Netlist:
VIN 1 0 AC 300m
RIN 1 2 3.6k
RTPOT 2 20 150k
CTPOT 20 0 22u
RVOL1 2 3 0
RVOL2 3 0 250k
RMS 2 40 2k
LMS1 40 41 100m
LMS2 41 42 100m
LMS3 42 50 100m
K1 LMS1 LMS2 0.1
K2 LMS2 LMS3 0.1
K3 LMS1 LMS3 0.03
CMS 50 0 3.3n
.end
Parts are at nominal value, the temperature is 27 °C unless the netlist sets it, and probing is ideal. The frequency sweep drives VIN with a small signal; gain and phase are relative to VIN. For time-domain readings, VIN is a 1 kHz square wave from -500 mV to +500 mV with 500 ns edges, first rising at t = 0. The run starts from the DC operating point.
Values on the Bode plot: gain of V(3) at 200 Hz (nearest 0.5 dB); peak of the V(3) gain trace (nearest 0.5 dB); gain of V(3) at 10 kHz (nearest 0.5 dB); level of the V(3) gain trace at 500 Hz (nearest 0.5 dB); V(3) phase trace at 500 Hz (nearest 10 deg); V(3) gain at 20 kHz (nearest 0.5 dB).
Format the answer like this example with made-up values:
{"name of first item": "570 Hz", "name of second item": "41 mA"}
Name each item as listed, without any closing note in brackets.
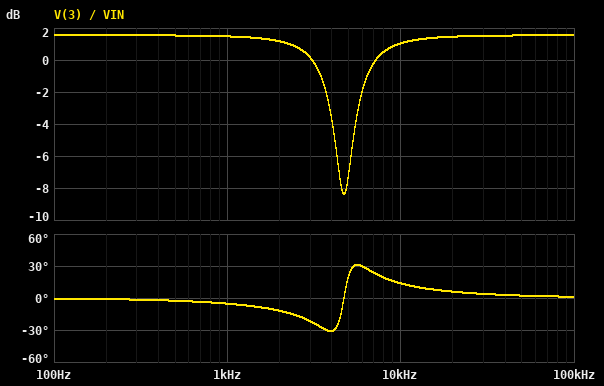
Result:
{"gain of V(3) at 200 Hz": "1.5 dB", "peak of the V(3) gain trace": "1.5 dB", "gain of V(3) at 10 kHz": "1.0 dB", "level of the V(3) gain trace at 500 Hz": "1.5 dB", "V(3) phase trace at 500 Hz": "0 deg", "V(3) gain at 20 kHz": "1.5 dB"}
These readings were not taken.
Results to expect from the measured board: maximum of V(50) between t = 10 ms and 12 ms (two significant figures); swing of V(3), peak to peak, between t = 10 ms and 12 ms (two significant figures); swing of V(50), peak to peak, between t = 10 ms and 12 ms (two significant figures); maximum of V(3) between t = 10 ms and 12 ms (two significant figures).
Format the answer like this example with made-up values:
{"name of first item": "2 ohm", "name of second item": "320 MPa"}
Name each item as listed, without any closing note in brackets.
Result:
{"maximum of V(50) between t = 10 ms and 12 ms": "1.0 V", "swing of V(3), peak to peak, between t = 10 ms and 12 ms": "1.4 V", "swing of V(50), peak to peak, between t = 10 ms and 12 ms": "2.1 V", "maximum of V(3) between t = 10 ms and 12 ms": "700 mV"}
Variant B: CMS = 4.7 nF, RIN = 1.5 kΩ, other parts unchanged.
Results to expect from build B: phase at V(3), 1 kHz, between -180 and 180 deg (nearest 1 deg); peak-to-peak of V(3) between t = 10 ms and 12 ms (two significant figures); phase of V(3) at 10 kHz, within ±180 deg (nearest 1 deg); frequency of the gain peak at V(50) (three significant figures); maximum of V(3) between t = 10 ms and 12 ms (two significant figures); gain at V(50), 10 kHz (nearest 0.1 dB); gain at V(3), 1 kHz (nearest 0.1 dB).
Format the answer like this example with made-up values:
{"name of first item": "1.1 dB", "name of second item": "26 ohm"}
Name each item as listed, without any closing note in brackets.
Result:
{"phase at V(3), 1 kHz, between -180 and 180 deg": "-3 deg", "peak-to-peak of V(3) between t = 10 ms and 12 ms": "1.3 V", "phase of V(3) at 10 kHz, within ±180 deg": "5 deg", "frequency of the gain peak at V(50)": "3.76 kHz", "maximum of V(3) between t = 10 ms and 12 ms": "630 mV", "gain at V(50), 10 kHz": "-13.9 dB", "gain at V(3), 1 kHz": "0.9 dB"}
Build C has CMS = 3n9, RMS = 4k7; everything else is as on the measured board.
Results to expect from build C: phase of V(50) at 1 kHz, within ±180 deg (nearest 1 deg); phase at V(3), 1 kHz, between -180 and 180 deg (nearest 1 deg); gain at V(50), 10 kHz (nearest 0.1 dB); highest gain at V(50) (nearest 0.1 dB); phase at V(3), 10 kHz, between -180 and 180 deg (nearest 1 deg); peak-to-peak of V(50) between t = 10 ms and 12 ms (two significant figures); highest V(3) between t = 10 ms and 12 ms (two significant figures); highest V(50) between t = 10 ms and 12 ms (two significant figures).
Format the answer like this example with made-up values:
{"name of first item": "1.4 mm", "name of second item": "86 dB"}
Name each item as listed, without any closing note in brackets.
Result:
{"phase of V(50) at 1 kHz, within ±180 deg": "-12 deg", "phase at V(3), 1 kHz, between -180 and 180 deg": "-5 deg", "gain at V(50), 10 kHz": "-13.5 dB", "highest gain at V(50)": "2.1 dB", "phase at V(3), 10 kHz, between -180 and 180 deg": "10 deg", "peak-to-peak of V(50) between t = 10 ms and 12 ms": "1.4 V", "highest V(3) between t = 10 ms and 12 ms": "540 mV", "highest V(50) between t = 10 ms and 12 ms": "710 mV"}
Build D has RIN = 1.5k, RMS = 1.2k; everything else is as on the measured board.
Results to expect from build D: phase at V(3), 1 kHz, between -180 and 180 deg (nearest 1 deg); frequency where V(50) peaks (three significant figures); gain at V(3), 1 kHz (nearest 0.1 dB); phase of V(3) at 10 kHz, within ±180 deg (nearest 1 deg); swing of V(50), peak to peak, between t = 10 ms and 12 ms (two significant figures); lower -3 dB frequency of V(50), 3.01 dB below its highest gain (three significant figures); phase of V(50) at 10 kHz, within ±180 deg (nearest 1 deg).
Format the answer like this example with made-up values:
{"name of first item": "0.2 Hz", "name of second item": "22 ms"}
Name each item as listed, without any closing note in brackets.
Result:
{"phase at V(3), 1 kHz, between -180 and 180 deg": "-2 deg", "frequency where V(50) peaks": "4.62 kHz", "gain at V(3), 1 kHz": "0.5 dB", "phase of V(3) at 10 kHz, within ±180 deg": "5 deg", "swing of V(50), peak to peak, between t = 10 ms and 12 ms": "2.5 V", "lower -3 dB frequency of V(50), 3.01 dB below its highest gain": "3.92 kHz", "phase of V(50) at 10 kHz, within ±180 deg": "-171 deg"}
